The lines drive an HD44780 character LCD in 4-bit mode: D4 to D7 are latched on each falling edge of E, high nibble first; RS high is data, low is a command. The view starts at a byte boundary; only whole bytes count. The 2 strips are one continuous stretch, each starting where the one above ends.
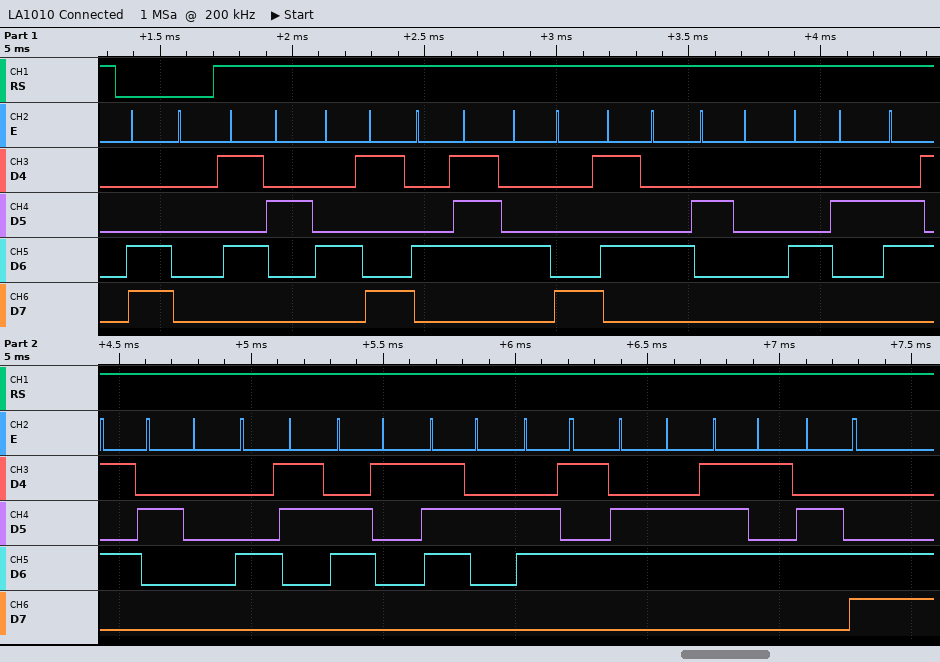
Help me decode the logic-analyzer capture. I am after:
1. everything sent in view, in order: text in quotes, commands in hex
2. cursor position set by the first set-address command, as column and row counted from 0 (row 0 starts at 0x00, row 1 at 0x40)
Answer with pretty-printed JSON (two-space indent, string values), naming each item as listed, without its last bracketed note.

{
  "everything sent in view, in order: text in quotes, commands in hex": "0xC0 \"RIGHT Be Careful\"",
  "cursor position set by the first set-address command, as column and row counted from 0": "column 0, row 1"
}
